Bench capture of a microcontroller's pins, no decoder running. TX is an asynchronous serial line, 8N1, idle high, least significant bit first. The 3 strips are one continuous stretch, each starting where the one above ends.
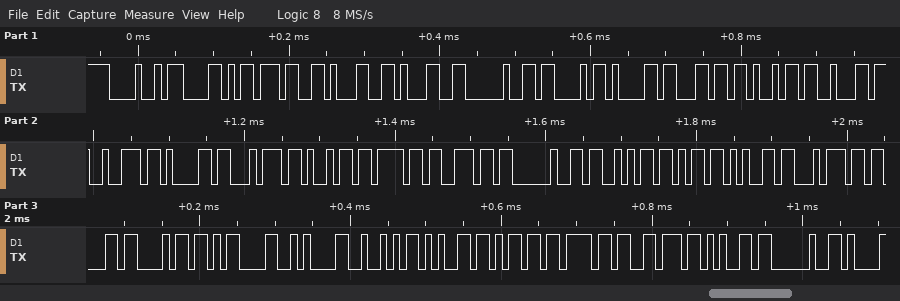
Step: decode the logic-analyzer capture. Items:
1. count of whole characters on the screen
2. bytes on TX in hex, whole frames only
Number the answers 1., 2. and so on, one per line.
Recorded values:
1. 33
2. 48 58 37 31 31 20 43 61 6C 69 62 72 61 74 69 6F 6E 20 53 6B 65 74 63 68 0D 0A 52 65 6D 6F 76 65 20
